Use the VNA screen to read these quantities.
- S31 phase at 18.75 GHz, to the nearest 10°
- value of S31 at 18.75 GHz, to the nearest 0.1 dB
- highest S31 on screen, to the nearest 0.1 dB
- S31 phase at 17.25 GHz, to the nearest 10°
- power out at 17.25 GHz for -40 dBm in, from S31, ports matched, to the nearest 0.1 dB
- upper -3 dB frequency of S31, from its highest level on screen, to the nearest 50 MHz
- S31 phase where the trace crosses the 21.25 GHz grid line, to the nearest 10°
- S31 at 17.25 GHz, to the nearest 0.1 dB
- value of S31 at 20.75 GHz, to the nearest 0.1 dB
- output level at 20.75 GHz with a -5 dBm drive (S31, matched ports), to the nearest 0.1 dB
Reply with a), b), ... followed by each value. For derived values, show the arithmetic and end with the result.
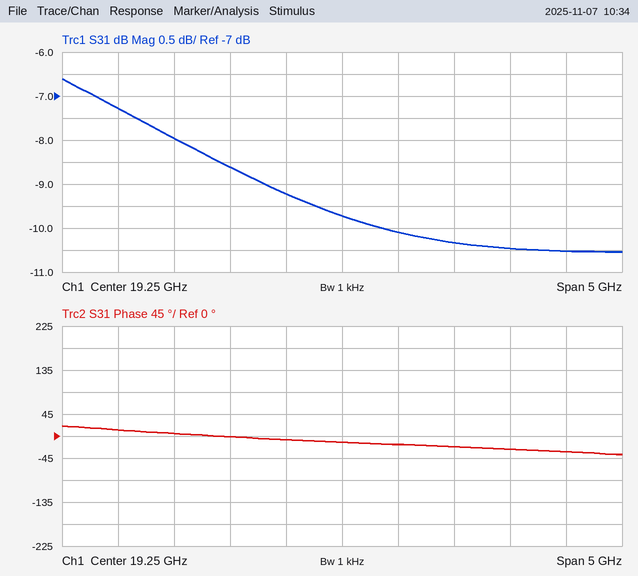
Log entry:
a) -10°
b) -9.2 dB
c) -6.6 dB
d) 10°
e) -40 dBm + (-7.3 dB) = -47.3 dBm
f) 19.15 GHz
g) -30°
h) -7.3 dB
i) -10.5 dB
j) -5 dBm + (-10.5 dB) = -15.5 dBm
